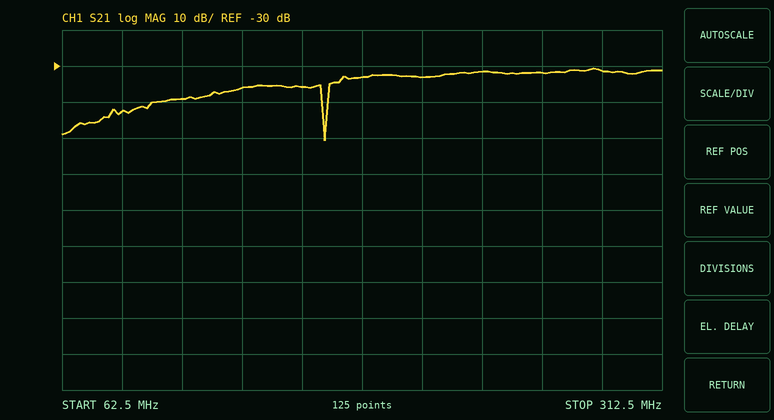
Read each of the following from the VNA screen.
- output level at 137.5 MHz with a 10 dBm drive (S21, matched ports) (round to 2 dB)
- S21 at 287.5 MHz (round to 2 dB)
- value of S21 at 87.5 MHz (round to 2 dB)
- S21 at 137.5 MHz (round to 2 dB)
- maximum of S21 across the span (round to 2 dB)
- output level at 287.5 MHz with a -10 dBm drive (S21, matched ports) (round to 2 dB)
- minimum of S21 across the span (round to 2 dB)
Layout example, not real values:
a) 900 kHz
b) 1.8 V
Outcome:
a) -26 dBm
b) -32 dB
c) -42 dB
d) -36 dB
e) -30 dB
f) -42 dBm
g) -50 dB
